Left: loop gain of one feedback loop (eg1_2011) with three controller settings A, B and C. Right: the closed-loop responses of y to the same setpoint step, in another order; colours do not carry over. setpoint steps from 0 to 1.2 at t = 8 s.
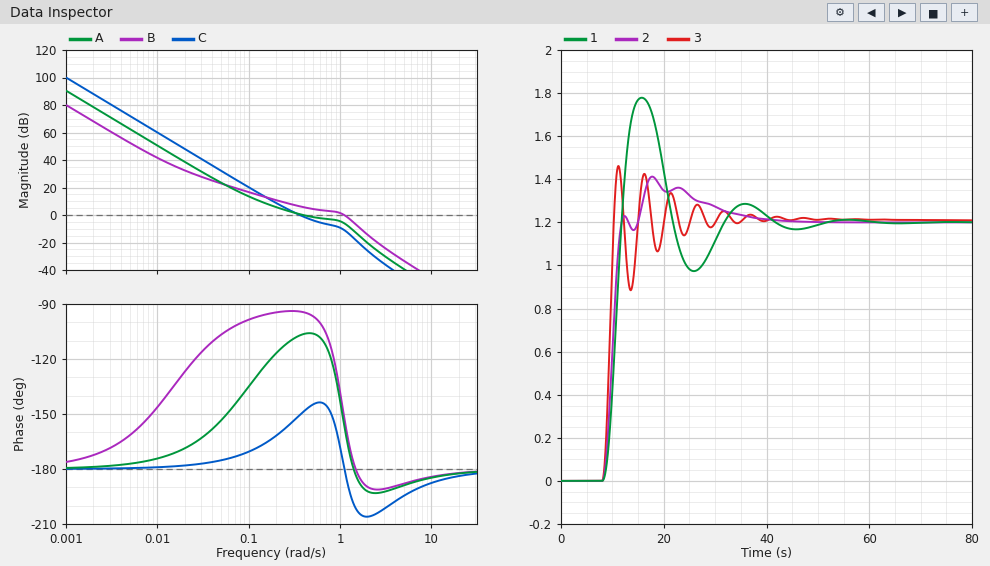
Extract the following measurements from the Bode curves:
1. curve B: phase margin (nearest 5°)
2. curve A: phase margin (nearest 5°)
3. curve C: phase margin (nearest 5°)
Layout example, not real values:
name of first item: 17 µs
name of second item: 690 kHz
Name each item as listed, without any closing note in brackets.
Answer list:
curve B: phase margin: 30°
curve A: phase margin: 75°
curve C: phase margin: 30°
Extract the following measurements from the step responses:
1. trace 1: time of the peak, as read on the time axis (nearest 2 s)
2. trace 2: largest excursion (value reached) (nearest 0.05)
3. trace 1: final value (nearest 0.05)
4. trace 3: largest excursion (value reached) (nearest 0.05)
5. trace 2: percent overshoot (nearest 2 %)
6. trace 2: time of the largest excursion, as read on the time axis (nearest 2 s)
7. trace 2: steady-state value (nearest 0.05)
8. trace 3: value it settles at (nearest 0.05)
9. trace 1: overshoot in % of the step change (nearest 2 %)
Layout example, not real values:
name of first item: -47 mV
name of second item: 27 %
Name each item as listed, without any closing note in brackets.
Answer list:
trace 1: time of the peak, as read on the time axis: 16 s
trace 2: largest excursion (value reached): 1.40
trace 1: final value: 1.20
trace 3: largest excursion (value reached): 1.45
trace 2: percent overshoot: 18 %
trace 2: time of the largest excursion, as read on the time axis: 18 s
trace 2: steady-state value: 1.20
trace 3: value it settles at: 1.20
trace 1: overshoot in % of the step change: 48 %
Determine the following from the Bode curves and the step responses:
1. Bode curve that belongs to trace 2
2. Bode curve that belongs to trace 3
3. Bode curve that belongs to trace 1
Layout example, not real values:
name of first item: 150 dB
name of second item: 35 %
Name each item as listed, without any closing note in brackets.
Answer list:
Bode curve that belongs to trace 2: A
Bode curve that belongs to trace 3: B
Bode curve that belongs to trace 1: C
